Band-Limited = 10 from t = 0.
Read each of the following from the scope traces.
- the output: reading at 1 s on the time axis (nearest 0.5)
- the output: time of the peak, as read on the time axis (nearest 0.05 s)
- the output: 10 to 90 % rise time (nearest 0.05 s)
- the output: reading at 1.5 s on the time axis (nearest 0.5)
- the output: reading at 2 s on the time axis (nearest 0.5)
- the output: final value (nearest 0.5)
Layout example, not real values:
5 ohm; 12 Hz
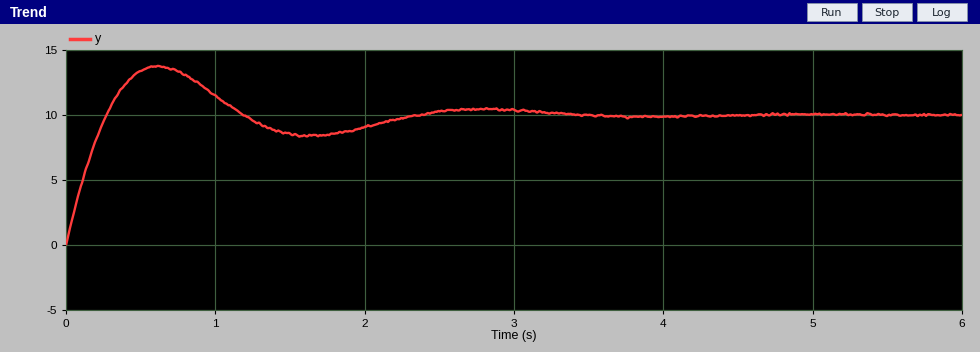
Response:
11.5; 0.60 s; 0.20 s; 8.5; 9.0; 10.0
